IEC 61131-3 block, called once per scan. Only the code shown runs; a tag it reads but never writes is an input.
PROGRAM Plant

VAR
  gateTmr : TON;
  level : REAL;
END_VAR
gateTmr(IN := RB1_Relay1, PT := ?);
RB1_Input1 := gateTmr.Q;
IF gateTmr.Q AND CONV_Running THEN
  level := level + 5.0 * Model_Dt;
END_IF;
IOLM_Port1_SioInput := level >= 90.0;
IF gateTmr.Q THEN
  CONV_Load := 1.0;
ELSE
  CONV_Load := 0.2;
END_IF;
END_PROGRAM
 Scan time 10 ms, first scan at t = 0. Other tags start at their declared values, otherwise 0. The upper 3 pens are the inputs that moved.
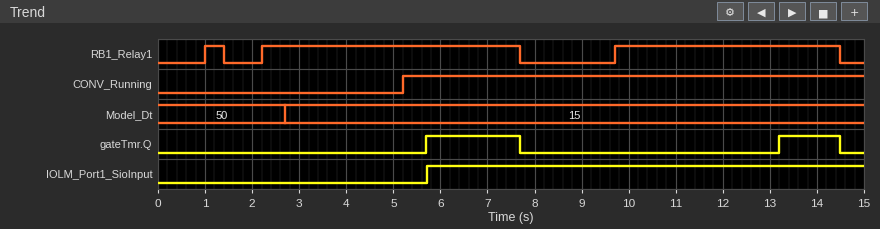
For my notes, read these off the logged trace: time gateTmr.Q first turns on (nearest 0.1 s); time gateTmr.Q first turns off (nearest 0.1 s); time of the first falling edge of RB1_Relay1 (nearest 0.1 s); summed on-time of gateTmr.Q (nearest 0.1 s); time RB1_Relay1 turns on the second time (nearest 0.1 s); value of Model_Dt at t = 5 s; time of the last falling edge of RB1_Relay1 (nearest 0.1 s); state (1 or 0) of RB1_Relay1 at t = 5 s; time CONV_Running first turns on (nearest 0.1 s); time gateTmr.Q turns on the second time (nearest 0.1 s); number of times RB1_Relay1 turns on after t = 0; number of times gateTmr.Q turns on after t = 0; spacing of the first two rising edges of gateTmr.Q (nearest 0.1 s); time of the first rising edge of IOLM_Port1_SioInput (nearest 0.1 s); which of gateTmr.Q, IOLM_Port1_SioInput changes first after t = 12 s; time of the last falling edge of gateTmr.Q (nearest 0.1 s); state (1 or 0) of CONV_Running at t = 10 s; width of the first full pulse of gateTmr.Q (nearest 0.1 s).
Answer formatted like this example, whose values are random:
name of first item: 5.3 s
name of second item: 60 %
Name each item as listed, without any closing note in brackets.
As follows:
time gateTmr.Q first turns on: 5.7 s
time gateTmr.Q first turns off: 7.7 s
time of the first falling edge of RB1_Relay1: 1.4 s
summed on-time of gateTmr.Q: 3.3 s
time RB1_Relay1 turns on the second time: 2.2 s
value of Model_Dt at t = 5 s: 15
time of the last falling edge of RB1_Relay1: 14.5 s
state (1 or 0) of RB1_Relay1 at t = 5 s: 1
time CONV_Running first turns on: 5.2 s
time gateTmr.Q turns on the second time: 13.2 s
number of times RB1_Relay1 turns on after t = 0: 3
number of times gateTmr.Q turns on after t = 0: 2
spacing of the first two rising edges of gateTmr.Q: 7.5 s
time of the first rising edge of IOLM_Port1_SioInput: 5.7 s
which of gateTmr.Q, IOLM_Port1_SioInput changes first after t = 12 s: gateTmr.Q
time of the last falling edge of gateTmr.Q: 14.5 s
state (1 or 0) of CONV_Running at t = 10 s: 1
width of the first full pulse of gateTmr.Q: 2.0 s
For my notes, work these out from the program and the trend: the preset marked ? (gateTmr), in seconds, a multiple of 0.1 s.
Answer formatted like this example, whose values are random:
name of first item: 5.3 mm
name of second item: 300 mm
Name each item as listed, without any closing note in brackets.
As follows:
the preset marked ? (gateTmr), in seconds, a multiple of 0.1 s: 3.5 s
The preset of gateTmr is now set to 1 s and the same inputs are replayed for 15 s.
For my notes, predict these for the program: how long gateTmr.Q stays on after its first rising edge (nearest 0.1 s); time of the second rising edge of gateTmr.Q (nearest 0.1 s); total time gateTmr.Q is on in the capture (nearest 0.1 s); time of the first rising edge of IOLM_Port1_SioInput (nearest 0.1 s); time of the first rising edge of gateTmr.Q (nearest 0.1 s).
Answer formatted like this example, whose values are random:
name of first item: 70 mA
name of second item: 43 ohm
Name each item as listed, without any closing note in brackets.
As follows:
how long gateTmr.Q stays on after its first rising edge: 4.5 s
time of the second rising edge of gateTmr.Q: 10.7 s
total time gateTmr.Q is on in the capture: 8.3 s
time of the first rising edge of IOLM_Port1_SioInput: 5.2 s
time of the first rising edge of gateTmr.Q: 3.2 s
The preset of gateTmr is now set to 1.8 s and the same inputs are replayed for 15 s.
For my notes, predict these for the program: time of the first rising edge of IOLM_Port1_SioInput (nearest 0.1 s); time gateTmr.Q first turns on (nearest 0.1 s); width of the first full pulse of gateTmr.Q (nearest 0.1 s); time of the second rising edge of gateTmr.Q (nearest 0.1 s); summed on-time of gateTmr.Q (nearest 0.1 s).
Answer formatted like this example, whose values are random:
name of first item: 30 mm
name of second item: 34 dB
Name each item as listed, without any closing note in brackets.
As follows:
time of the first rising edge of IOLM_Port1_SioInput: 5.2 s
time gateTmr.Q first turns on: 4.0 s
width of the first full pulse of gateTmr.Q: 3.7 s
time of the second rising edge of gateTmr.Q: 11.5 s
summed on-time of gateTmr.Q: 6.7 s
